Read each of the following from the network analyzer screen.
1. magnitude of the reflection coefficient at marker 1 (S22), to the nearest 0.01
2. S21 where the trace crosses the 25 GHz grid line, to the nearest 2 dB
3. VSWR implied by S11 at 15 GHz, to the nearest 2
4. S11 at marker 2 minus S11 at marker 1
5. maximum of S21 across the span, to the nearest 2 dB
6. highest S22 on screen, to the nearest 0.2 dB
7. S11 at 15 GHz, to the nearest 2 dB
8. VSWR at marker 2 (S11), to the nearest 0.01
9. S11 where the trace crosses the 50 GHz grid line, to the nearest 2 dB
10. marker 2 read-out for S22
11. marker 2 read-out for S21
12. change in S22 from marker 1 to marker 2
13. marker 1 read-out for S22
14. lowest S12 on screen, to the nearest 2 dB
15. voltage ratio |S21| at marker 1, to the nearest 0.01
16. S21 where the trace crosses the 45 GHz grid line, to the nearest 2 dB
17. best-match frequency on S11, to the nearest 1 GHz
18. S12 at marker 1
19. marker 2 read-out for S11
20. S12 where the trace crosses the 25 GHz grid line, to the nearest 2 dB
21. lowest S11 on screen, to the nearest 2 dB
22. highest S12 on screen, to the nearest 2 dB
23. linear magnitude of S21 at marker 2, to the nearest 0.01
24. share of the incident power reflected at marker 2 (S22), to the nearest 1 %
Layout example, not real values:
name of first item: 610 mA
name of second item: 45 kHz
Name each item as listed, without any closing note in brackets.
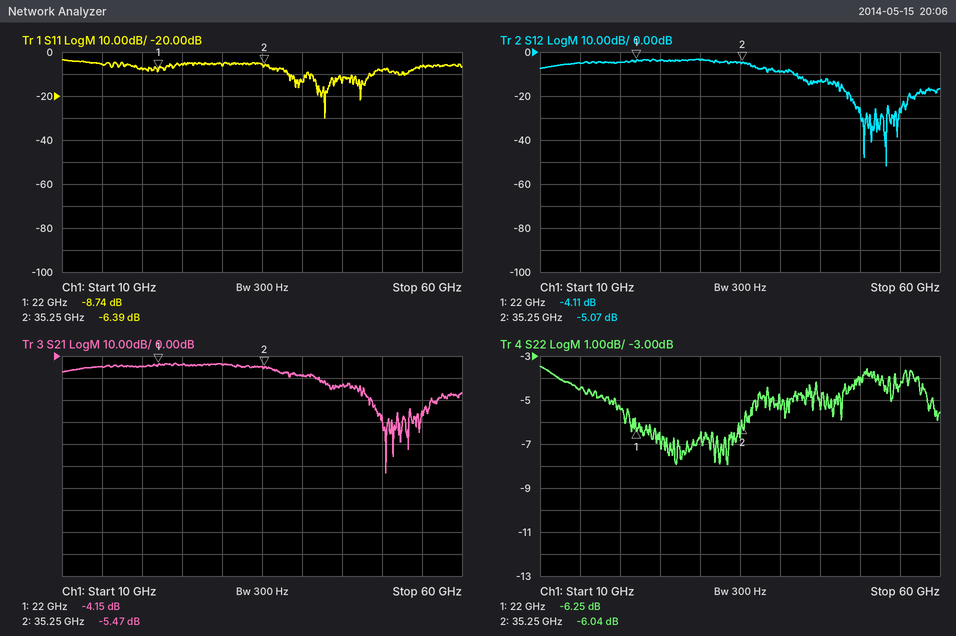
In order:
magnitude of the reflection coefficient at marker 1 (S22), to the nearest 0.01: 0.49
S21 where the trace crosses the 25 GHz grid line, to the nearest 2 dB: -4 dB
VSWR implied by S11 at 15 GHz, to the nearest 2: 4
S11 at marker 2 minus S11 at marker 1: 2.35 dB
maximum of S21 across the span, to the nearest 2 dB: -4 dB
highest S22 on screen, to the nearest 0.2 dB: -3.4 dB
S11 at 15 GHz, to the nearest 2 dB: -6 dB
VSWR at marker 2 (S11), to the nearest 0.01: 2.84
S11 where the trace crosses the 50 GHz grid line, to the nearest 2 dB: -8 dB
marker 2 read-out for S22: -6.04 dB
marker 2 read-out for S21: -5.47 dB
change in S22 from marker 1 to marker 2: 0.21 dB
marker 1 read-out for S22: -6.25 dB
lowest S12 on screen, to the nearest 2 dB: -52 dB
voltage ratio |S21| at marker 1, to the nearest 0.01: 0.62
S21 where the trace crosses the 45 GHz grid line, to the nearest 2 dB: -14 dB
best-match frequency on S11, to the nearest 1 GHz: 43 GHz
S12 at marker 1: -4.11 dB
marker 2 read-out for S11: -6.39 dB
S12 where the trace crosses the 25 GHz grid line, to the nearest 2 dB: -4 dB
lowest S11 on screen, to the nearest 2 dB: -30 dB
highest S12 on screen, to the nearest 2 dB: -4 dB
linear magnitude of S21 at marker 2, to the nearest 0.01: 0.53
share of the incident power reflected at marker 2 (S22), to the nearest 1 %: 25 %
